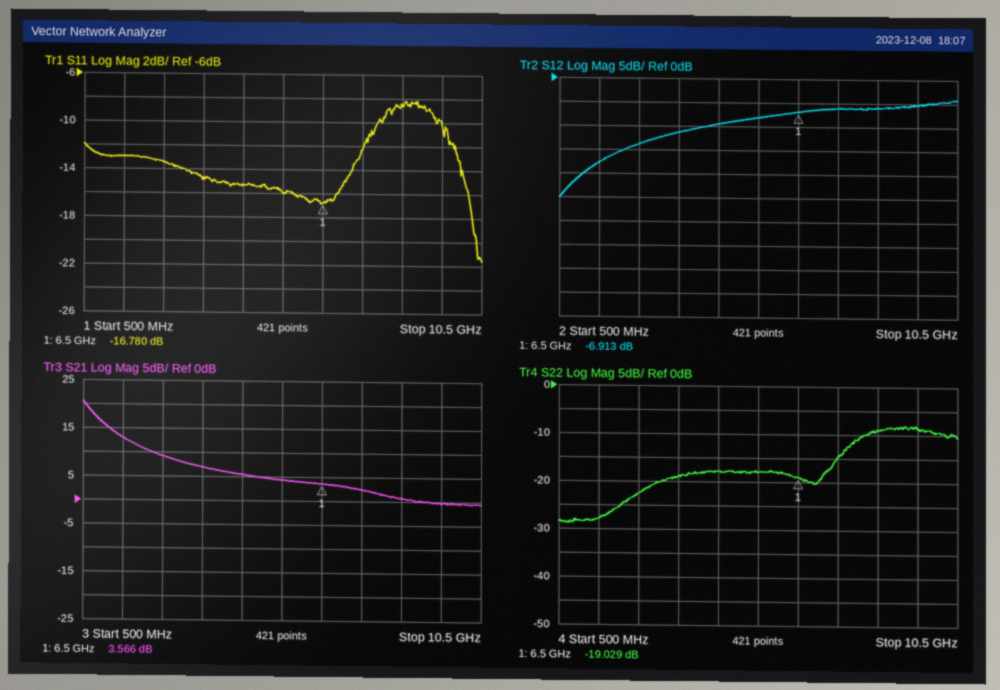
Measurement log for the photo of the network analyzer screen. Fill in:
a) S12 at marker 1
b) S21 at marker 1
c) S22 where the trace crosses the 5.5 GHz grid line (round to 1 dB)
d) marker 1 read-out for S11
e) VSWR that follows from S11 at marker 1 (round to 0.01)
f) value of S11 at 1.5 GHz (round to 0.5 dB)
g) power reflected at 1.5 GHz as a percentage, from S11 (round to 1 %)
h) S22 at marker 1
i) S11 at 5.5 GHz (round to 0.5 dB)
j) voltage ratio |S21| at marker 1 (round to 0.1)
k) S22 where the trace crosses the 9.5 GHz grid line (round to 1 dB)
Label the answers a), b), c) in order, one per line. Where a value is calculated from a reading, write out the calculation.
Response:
a) -6.913 dB
b) 3.566 dB
c) -18 dB
d) -16.780 dB
e) (1 + 0.1449)/(1 − 0.1449) ≈ 1.34
f) -13.0 dB
g) 10^(-13/10) ≈ 5 %
h) -19.029 dB
i) -16.0 dB
j) 10^(3.566/20) ≈ 1.5
k) -9 dB
